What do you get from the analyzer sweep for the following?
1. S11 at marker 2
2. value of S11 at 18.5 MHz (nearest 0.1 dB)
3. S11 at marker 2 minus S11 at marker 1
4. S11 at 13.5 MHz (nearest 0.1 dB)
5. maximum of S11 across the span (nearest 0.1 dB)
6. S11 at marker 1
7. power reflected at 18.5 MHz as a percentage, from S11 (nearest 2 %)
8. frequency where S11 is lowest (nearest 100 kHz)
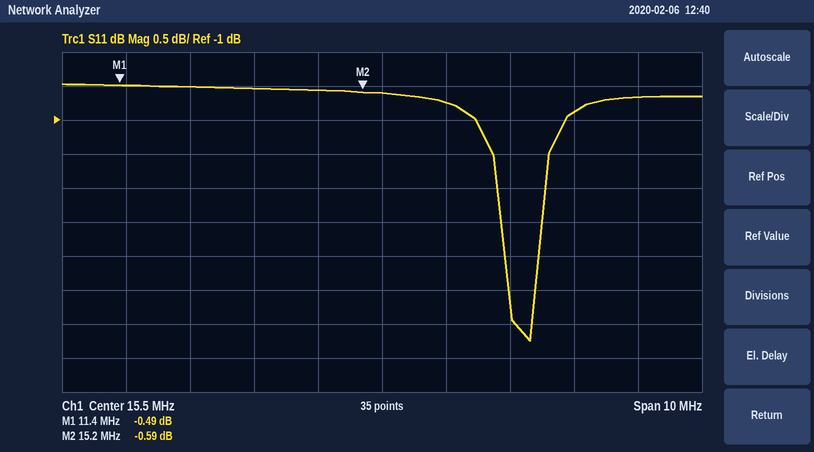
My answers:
-0.59 dB
-0.9 dB
-0.10 dB
-0.5 dB
-0.5 dB
-0.49 dB
82 %
17.8 MHz
